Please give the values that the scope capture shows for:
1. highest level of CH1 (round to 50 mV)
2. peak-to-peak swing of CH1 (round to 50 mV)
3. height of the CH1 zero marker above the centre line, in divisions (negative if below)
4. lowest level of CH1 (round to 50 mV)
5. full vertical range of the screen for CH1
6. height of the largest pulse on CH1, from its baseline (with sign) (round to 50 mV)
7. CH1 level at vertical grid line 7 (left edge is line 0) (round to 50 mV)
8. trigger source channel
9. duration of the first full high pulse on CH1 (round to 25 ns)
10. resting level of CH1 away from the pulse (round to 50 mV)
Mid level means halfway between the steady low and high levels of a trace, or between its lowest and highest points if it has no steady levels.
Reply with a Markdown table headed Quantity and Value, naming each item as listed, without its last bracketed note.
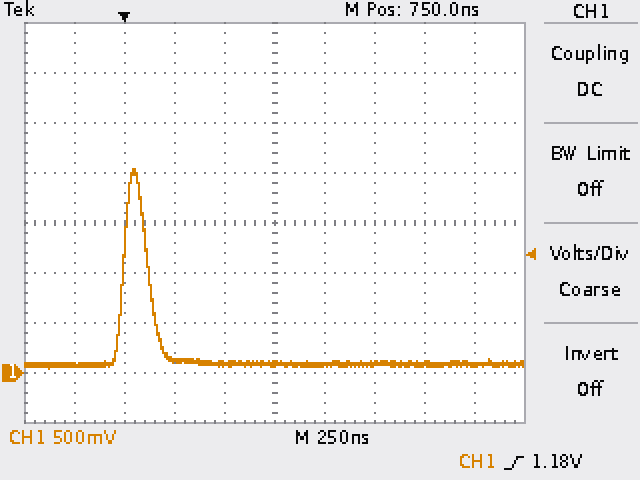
| Quantity | Value |
|---|---|
| highest level of CH1 | 2.05 V |
| peak-to-peak swing of CH1 | 2.00 V |
| height of the CH1 zero marker above the centre line, in divisions | -3.0 div |
| lowest level of CH1 | 50 mV |
| full vertical range of the screen for CH1 | 4 V |
| height of the largest pulse on CH1, from its baseline (with sign) | +1.95 V |
| CH1 level at vertical grid line 7 (left edge is line 0) | 100 mV |
| trigger source channel | CH1 |
| duration of the first full high pulse on CH1 | 125 ns |
| resting level of CH1 away from the pulse | 100 mV |
